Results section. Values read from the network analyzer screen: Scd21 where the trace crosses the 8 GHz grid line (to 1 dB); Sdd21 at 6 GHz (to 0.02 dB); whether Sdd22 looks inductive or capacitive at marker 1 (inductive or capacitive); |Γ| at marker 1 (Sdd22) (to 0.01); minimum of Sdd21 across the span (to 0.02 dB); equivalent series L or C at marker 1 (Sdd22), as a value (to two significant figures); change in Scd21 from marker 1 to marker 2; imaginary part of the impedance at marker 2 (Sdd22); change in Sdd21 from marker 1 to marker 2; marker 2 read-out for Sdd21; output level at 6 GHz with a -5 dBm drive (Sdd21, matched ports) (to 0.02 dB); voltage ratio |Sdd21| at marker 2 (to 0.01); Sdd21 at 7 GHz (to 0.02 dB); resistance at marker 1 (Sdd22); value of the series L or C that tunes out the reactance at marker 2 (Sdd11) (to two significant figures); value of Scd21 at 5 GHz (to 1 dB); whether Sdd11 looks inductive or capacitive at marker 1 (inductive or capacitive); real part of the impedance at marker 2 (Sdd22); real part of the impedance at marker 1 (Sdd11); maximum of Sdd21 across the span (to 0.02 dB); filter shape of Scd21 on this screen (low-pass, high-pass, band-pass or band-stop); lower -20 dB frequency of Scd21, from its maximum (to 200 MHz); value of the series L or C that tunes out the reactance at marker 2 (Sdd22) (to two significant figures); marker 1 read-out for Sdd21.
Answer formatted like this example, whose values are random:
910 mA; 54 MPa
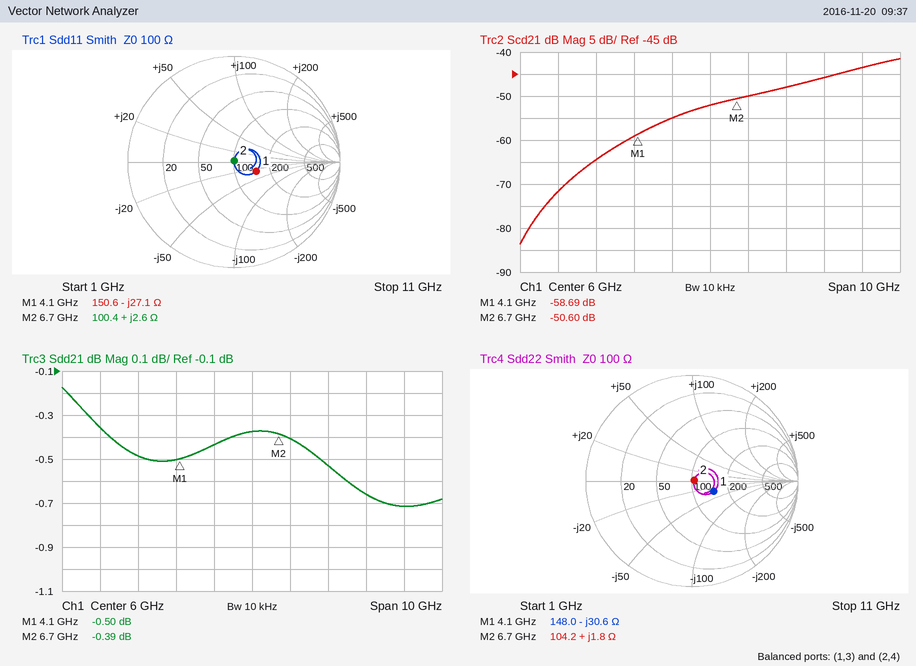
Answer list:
-48 dB; -0.38 dB; capacitive; 0.23; -0.72 dB; 1.3 pF; 8.09 dB; +1.8 Ω; 0.11 dB; -0.39 dB; -5.38 dBm; 0.96; -0.40 dB; 148.0 Ω; 9.1 pF; -55 dB; capacitive; 104.2 Ω; 150.6 Ω; -0.18 dB; high-pass; 3.6 GHz; 13 pF; -0.50 dB
